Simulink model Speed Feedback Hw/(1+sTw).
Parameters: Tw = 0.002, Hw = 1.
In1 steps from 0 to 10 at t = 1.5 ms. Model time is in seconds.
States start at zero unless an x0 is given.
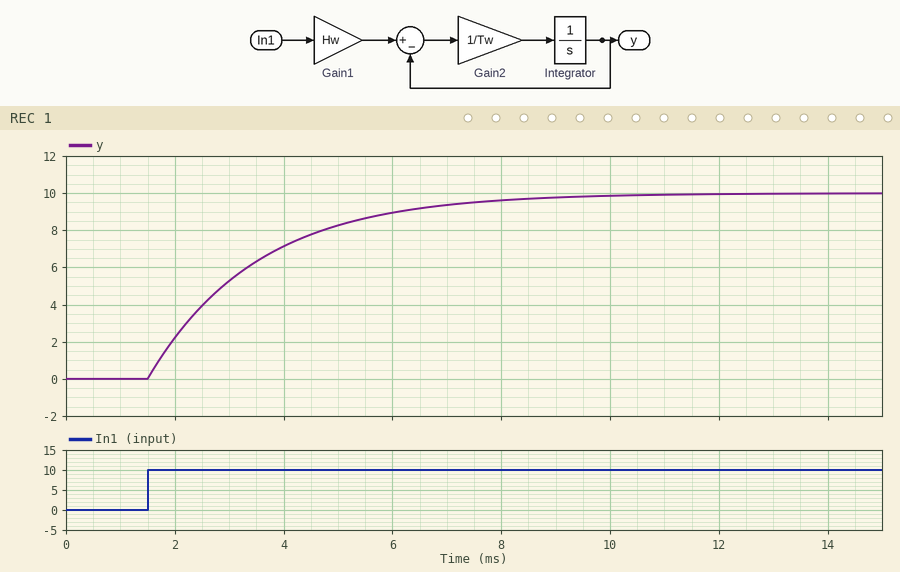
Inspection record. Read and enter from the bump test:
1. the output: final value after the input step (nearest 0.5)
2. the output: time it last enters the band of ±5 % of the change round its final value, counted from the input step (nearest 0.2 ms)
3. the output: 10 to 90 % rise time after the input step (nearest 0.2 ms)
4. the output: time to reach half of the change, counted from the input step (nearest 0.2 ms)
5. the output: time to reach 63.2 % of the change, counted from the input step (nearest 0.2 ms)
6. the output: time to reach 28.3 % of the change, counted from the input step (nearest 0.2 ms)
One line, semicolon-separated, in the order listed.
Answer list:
10.0; 6.0 ms; 4.4 ms; 1.4 ms; 2.0 ms; 0.6 ms
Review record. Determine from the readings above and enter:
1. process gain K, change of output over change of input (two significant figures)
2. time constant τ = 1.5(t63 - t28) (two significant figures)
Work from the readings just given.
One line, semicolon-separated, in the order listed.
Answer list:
1.0; 2.1 ms
